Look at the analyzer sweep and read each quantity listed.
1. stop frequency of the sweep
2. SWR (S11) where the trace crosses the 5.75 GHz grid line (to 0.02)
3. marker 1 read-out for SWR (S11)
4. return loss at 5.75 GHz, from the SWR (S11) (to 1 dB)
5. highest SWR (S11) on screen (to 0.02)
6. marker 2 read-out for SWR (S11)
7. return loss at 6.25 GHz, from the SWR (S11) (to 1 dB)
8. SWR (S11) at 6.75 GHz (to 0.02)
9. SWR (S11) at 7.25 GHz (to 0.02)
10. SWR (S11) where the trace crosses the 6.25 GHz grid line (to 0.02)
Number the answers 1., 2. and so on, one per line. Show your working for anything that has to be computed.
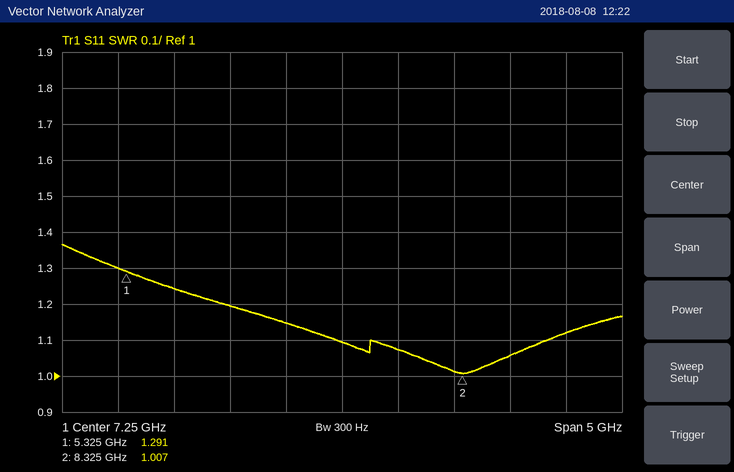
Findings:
1. 9.75 GHz
2. 1.24
3. 1.291
4. −20 log10((1.24 − 1)/(1.24 + 1)) ≈ 19 dB
5. 1.36
6. 1.007
7. −20 log10((1.2 − 1)/(1.2 + 1)) ≈ 21 dB
8. 1.14
9. 1.10
10. 1.20
